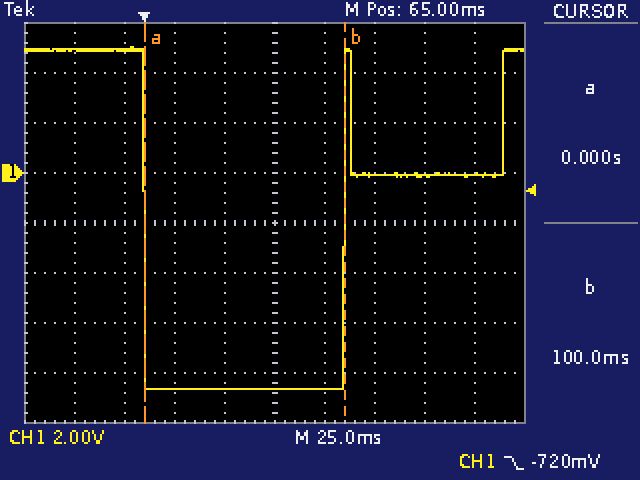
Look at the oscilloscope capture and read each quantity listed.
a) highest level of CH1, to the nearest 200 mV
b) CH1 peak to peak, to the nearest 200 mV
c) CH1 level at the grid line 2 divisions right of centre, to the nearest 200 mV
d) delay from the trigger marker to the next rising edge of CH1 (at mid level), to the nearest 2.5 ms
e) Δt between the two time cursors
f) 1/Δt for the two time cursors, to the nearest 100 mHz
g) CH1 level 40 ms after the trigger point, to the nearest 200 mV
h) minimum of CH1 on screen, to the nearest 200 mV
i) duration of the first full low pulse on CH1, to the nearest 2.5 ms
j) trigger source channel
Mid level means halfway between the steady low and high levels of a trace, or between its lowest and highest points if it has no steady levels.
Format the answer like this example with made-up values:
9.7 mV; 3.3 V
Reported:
5.0 V; 13.6 V; 0.0 V; 100.0 ms; 100.0 ms; 10.0 Hz; -8.6 V; -8.6 V; 100.0 ms; CH1
